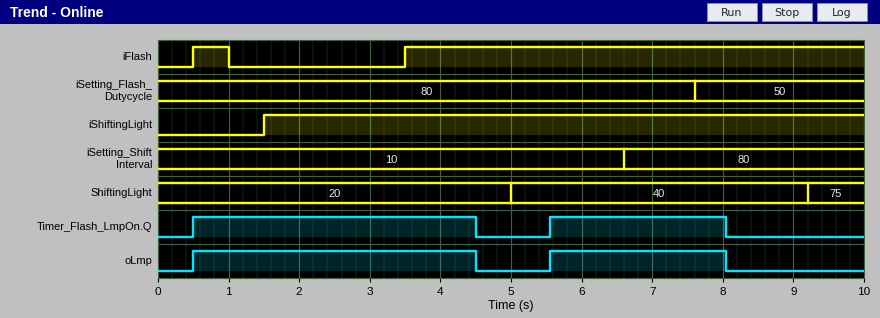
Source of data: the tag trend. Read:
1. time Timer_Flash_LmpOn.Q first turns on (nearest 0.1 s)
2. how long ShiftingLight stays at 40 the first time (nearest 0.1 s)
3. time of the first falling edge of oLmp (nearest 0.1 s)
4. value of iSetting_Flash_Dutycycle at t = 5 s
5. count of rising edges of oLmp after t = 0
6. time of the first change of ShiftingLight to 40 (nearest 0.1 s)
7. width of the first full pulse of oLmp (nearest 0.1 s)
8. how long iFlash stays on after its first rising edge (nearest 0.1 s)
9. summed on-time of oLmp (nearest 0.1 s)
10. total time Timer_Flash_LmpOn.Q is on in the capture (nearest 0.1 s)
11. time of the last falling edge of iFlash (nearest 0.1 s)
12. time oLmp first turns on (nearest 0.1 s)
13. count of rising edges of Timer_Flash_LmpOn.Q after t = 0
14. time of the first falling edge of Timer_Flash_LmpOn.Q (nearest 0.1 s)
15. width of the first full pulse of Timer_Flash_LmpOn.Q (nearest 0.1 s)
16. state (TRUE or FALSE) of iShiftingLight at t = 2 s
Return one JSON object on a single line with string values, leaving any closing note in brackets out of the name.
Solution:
{"time Timer_Flash_LmpOn.Q first turns on": "0.5 s", "how long ShiftingLight stays at 40 the first time": "4.2 s", "time of the first falling edge of oLmp": "4.5 s", "value of iSetting_Flash_Dutycycle at t = 5 s": "80", "count of rising edges of oLmp after t = 0": "2", "time of the first change of ShiftingLight to 40": "5.0 s", "width of the first full pulse of oLmp": "4.0 s", "how long iFlash stays on after its first rising edge": "0.5 s", "summed on-time of oLmp": "6.5 s", "total time Timer_Flash_LmpOn.Q is on in the capture": "6.5 s", "time of the last falling edge of iFlash": "1.0 s", "time oLmp first turns on": "0.5 s", "count of rising edges of Timer_Flash_LmpOn.Q after t = 0": "2", "time of the first falling edge of Timer_Flash_LmpOn.Q": "4.5 s", "width of the first full pulse of Timer_Flash_LmpOn.Q": "4.0 s", "state (TRUE or FALSE) of iShiftingLight at t = 2 s": "TRUE"}
